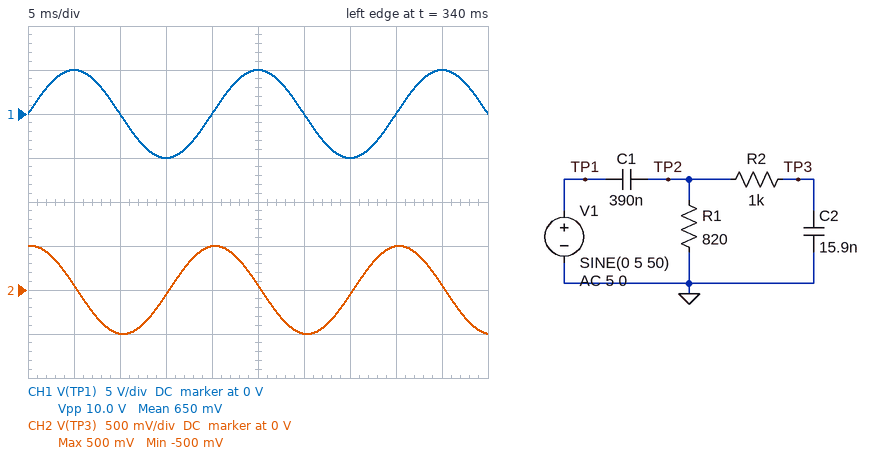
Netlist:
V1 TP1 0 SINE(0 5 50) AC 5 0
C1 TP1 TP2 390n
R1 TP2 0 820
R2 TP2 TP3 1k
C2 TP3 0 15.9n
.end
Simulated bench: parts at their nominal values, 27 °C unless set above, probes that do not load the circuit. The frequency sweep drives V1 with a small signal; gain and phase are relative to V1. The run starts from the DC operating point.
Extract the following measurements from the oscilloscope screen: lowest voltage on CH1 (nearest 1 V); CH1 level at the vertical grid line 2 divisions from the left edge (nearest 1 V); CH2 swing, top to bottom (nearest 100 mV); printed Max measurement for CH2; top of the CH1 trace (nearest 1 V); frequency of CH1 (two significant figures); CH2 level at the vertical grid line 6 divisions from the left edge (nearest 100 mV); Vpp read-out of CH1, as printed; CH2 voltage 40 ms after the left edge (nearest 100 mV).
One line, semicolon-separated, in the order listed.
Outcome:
-5 V; 0 V; 1.0 V; 500 mV; 5 V; 50 Hz; -500 mV; 10.0 V; 500 mV
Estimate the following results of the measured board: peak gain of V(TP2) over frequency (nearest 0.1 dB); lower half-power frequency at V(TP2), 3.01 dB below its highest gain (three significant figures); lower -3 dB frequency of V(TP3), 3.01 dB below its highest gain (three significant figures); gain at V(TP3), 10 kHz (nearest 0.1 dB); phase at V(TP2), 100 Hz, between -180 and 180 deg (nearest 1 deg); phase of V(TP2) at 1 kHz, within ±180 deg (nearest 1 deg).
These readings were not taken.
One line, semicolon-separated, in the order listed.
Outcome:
0 dB; 521 Hz; 439 Hz; -3.2 dB; 78 deg; 26 deg
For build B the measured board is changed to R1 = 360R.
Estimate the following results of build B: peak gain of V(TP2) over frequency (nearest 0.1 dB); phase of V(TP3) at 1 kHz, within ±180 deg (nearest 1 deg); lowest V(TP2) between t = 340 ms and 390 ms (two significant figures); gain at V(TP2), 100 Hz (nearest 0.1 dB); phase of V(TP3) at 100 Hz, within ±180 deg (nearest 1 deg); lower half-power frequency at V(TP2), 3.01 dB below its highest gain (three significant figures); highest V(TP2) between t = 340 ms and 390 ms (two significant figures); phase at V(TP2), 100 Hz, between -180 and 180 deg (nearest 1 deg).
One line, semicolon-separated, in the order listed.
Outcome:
0 dB; 42 deg; -220 mV; -21.1 dB; 84 deg; 1.19 kHz; 220 mV; 85 deg
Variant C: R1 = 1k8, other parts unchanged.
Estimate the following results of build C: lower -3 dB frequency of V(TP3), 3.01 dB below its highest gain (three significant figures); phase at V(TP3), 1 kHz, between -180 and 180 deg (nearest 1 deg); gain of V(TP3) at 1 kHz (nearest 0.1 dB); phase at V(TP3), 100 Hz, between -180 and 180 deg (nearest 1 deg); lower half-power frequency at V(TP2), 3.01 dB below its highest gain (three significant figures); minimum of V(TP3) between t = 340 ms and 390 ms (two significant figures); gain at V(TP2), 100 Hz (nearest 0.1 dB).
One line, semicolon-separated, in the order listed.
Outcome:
209 Hz; 7 deg; -0.6 dB; 65 deg; 237 Hz; -1.1 V; -7.9 dB
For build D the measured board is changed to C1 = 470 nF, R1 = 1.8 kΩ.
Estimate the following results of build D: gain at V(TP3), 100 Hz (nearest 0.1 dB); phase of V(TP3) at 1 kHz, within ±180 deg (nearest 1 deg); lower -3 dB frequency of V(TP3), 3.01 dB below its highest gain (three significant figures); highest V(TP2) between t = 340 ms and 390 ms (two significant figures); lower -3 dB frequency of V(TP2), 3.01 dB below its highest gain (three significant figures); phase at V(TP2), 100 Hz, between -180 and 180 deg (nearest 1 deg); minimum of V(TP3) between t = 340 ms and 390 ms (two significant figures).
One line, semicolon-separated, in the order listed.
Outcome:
-6.6 dB; 5 deg; 176 Hz; 1.3 V; 195 Hz; 61 deg; -1.3 V
